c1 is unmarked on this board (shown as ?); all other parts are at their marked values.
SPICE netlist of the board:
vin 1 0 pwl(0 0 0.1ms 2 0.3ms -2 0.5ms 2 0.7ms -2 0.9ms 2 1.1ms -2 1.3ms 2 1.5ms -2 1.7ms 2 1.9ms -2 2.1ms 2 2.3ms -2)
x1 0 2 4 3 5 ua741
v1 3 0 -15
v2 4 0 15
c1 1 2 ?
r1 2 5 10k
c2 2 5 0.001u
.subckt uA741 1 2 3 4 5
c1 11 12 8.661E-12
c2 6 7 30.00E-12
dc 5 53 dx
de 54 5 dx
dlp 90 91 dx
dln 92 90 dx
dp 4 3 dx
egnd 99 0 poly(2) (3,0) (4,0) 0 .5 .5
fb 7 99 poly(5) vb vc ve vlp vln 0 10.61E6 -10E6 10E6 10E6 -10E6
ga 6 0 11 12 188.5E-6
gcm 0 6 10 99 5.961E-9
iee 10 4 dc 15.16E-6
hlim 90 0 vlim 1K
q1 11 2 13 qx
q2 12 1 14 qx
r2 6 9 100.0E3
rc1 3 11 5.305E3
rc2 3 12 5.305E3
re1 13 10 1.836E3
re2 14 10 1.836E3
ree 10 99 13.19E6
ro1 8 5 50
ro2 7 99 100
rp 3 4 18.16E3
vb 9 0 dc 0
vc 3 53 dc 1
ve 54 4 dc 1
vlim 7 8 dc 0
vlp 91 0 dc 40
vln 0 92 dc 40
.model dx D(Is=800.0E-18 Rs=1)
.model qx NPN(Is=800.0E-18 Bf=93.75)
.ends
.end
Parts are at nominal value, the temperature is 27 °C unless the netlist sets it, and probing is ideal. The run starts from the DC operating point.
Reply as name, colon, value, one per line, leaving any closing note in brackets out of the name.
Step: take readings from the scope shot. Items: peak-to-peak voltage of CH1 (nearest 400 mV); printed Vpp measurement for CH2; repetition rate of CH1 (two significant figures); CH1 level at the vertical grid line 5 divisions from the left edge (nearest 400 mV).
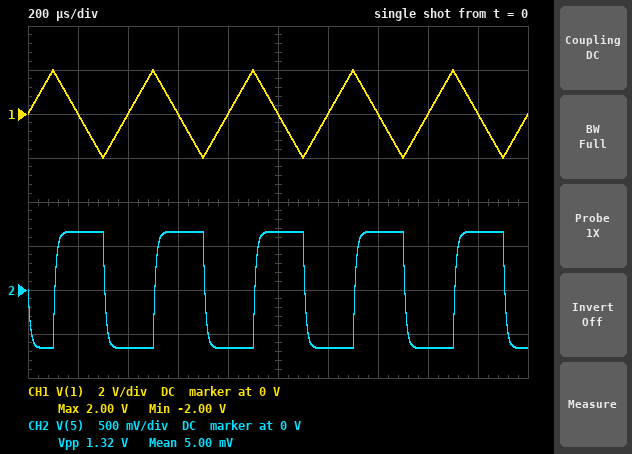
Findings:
peak-to-peak voltage of CH1: 4.0 V
printed Vpp measurement for CH2: 1.32 V
repetition rate of CH1: 2.5 kHz
CH1 level at the vertical grid line 5 divisions from the left edge: 0 V
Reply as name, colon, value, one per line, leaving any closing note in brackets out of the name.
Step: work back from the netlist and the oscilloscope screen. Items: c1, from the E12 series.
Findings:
c1, from the E12 series: 3.3 nF
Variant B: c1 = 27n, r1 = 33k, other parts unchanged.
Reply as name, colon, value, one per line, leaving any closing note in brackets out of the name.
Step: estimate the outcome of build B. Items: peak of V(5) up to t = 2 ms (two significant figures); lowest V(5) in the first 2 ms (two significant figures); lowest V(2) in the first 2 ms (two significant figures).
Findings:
peak of V(5) up to t = 2 ms: 15 V
lowest V(5) in the first 2 ms: -15 V
lowest V(2) in the first 2 ms: -580 mV
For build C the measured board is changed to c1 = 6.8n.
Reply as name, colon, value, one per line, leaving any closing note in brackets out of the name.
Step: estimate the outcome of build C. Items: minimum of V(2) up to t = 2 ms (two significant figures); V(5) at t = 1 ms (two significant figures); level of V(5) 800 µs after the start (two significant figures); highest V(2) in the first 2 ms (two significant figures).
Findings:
minimum of V(2) up to t = 2 ms: -37 mV
V(5) at t = 1 ms: 1.4 V
level of V(5) 800 µs after the start: -1.4 V
highest V(2) in the first 2 ms: 37 mV
